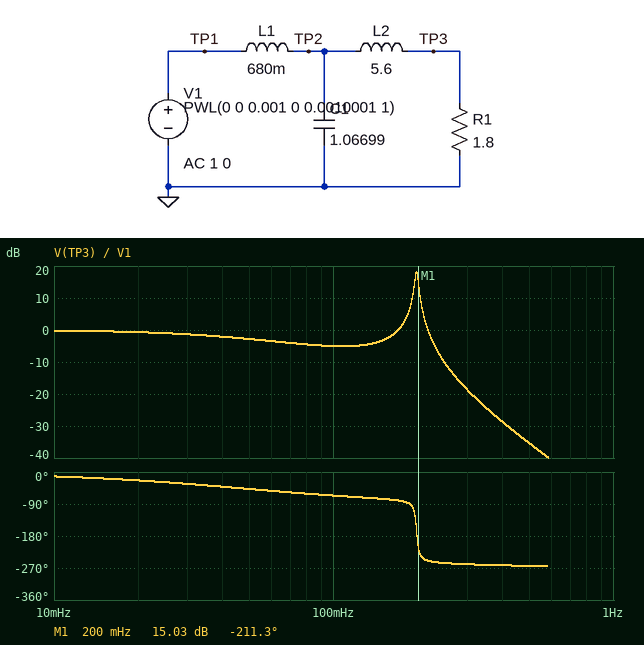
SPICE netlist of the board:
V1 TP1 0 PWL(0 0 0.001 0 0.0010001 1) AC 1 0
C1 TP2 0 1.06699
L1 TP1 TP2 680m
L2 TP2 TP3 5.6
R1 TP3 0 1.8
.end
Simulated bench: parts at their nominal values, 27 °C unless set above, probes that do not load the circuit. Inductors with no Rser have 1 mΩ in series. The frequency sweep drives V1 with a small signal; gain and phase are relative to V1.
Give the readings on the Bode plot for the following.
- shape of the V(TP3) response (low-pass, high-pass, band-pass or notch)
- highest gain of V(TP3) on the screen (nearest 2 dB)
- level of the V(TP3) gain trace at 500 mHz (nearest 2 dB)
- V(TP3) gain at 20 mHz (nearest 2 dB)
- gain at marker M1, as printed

band-pass
18 dB
-36 dB
0 dB
15.03 dB
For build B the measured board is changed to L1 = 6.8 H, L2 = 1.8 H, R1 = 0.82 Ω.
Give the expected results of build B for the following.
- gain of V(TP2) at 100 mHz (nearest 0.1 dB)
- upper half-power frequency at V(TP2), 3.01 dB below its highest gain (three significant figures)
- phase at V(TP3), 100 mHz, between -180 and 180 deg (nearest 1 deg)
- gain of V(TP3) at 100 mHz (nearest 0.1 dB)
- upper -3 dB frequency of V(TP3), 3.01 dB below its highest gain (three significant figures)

-5.6 dB
17.6 mHz
-125 deg
-10.2 dB
16.6 mHz
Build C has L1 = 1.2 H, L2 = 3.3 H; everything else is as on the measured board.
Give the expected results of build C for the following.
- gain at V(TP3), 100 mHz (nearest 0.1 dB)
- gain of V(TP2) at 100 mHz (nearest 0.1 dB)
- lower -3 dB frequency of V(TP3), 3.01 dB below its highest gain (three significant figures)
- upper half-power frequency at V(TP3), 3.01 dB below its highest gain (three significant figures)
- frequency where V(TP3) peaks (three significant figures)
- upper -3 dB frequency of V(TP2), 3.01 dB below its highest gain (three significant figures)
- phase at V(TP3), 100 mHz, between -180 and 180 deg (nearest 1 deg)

-0.9 dB
2.8 dB
148 mHz
168 mHz
159 mHz
169 mHz
-63 deg
